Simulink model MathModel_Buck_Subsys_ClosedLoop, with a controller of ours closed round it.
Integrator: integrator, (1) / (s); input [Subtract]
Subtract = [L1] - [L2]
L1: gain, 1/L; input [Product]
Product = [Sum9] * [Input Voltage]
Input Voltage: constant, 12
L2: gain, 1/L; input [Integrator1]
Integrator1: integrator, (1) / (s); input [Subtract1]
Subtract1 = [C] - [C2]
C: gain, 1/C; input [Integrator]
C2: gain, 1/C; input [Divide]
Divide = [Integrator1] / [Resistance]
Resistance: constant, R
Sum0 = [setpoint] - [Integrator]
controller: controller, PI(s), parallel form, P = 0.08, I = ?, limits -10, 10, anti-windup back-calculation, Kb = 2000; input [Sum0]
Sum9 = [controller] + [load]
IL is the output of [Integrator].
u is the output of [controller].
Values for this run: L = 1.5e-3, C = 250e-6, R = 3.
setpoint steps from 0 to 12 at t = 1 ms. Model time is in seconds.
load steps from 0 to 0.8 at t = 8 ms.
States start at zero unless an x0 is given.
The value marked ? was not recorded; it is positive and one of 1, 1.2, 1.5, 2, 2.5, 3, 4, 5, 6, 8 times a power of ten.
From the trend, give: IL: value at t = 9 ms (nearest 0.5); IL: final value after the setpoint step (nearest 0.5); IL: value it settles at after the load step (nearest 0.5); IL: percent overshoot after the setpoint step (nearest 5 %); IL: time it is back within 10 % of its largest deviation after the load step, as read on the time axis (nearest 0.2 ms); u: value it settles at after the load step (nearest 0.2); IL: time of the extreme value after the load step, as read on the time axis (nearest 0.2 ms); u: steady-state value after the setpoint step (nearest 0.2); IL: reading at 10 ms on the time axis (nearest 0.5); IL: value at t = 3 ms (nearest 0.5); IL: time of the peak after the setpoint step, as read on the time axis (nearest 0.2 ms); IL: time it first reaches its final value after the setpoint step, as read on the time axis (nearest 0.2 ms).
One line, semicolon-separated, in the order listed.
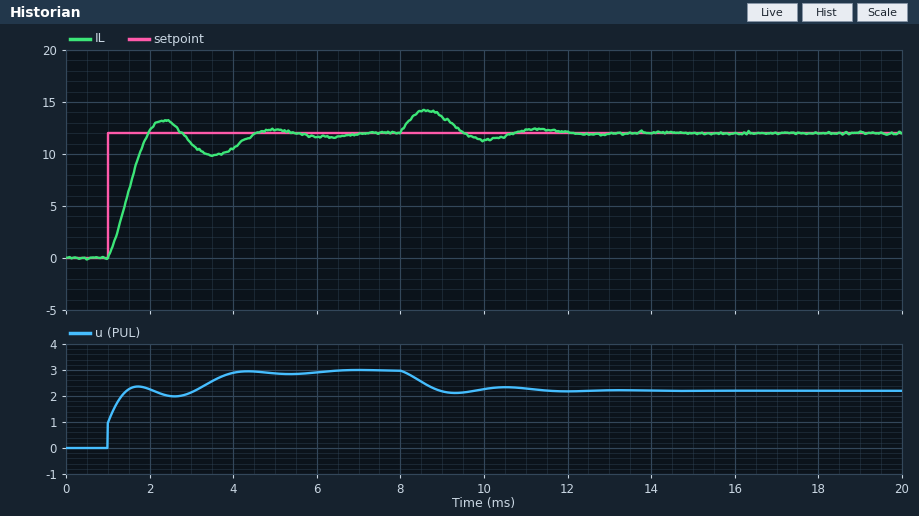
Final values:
13.5; 12.0; 12.0; 10 %; 11.8 ms; 2.2; 8.6 ms; 3.0; 11.5; 11.0; 2.4 ms; 2.0 ms
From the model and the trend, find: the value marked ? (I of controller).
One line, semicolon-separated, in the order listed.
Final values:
400
